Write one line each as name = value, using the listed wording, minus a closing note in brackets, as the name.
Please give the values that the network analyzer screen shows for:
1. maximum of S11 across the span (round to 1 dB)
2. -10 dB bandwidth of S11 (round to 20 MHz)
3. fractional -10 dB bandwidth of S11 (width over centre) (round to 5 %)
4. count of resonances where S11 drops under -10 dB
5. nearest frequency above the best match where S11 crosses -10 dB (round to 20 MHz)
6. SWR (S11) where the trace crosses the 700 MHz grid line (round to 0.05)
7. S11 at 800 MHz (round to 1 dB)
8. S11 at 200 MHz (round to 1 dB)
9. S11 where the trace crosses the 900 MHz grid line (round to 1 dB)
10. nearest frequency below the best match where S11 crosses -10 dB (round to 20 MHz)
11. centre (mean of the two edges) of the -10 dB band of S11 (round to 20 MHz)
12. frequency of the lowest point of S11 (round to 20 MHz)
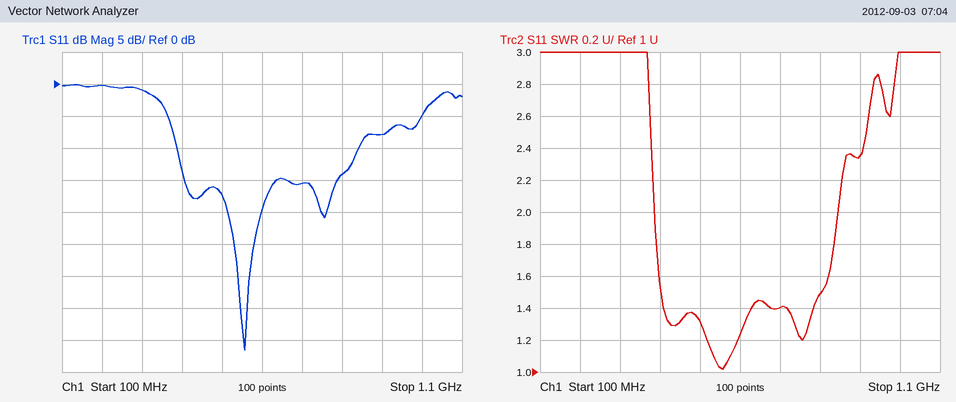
maximum of S11 across the span = 0 dB
-10 dB bandwidth of S11 = 460 MHz
fractional -10 dB bandwidth of S11 (width over centre) = 75 %
count of resonances where S11 drops under -10 dB = 2
nearest frequency above the best match where S11 crosses -10 dB = 840 MHz
SWR (S11) where the trace crosses the 700 MHz grid line = 1.40
S11 at 800 MHz = -14 dB
S11 at 200 MHz = 0 dB
S11 where the trace crosses the 900 MHz grid line = -8 dB
nearest frequency below the best match where S11 crosses -10 dB = 380 MHz
centre (mean of the two edges) of the -10 dB band of S11 = 620 MHz
frequency of the lowest point of S11 = 560 MHz
